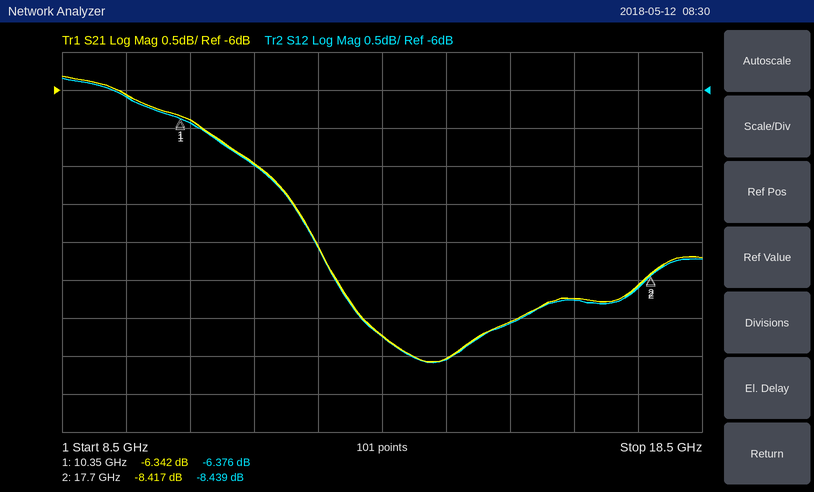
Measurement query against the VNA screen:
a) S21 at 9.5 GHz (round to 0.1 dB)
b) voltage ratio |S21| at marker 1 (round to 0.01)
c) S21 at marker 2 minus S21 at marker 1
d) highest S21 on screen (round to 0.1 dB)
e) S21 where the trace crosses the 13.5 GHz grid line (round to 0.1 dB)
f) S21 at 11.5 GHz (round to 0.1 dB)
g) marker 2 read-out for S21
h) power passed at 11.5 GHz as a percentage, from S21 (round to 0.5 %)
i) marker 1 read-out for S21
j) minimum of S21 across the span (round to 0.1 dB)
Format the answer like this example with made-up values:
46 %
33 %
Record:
-6.1 dB
0.48
-2.075 dB
-5.8 dB
-9.2 dB
-7.0 dB
-8.417 dB
20.0 %
-6.342 dB
-9.6 dB
